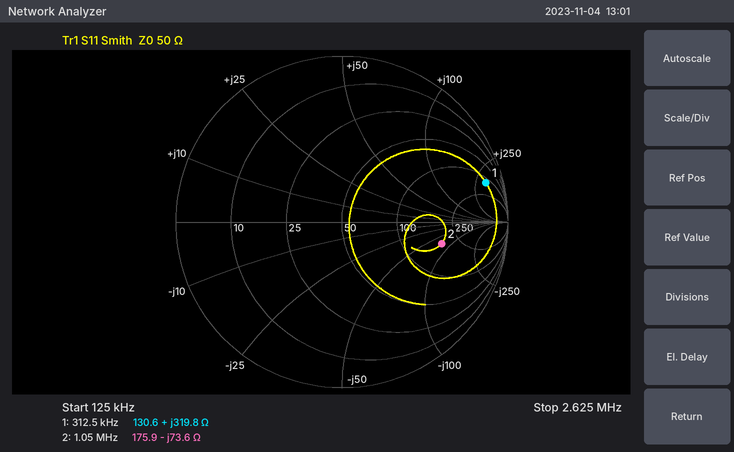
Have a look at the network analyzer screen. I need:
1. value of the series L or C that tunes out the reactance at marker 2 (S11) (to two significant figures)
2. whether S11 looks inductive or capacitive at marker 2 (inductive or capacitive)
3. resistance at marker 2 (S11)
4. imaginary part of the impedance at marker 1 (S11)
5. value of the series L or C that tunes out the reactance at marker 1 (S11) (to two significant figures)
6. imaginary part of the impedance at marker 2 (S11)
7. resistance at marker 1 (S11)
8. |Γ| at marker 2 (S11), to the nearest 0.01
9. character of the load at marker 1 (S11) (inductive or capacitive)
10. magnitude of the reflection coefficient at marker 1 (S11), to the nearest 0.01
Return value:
11 µH
capacitive
175.9 Ω
+319.8 Ω
1.6 nF
-73.6 Ω
130.6 Ω
0.61
inductive
0.90
